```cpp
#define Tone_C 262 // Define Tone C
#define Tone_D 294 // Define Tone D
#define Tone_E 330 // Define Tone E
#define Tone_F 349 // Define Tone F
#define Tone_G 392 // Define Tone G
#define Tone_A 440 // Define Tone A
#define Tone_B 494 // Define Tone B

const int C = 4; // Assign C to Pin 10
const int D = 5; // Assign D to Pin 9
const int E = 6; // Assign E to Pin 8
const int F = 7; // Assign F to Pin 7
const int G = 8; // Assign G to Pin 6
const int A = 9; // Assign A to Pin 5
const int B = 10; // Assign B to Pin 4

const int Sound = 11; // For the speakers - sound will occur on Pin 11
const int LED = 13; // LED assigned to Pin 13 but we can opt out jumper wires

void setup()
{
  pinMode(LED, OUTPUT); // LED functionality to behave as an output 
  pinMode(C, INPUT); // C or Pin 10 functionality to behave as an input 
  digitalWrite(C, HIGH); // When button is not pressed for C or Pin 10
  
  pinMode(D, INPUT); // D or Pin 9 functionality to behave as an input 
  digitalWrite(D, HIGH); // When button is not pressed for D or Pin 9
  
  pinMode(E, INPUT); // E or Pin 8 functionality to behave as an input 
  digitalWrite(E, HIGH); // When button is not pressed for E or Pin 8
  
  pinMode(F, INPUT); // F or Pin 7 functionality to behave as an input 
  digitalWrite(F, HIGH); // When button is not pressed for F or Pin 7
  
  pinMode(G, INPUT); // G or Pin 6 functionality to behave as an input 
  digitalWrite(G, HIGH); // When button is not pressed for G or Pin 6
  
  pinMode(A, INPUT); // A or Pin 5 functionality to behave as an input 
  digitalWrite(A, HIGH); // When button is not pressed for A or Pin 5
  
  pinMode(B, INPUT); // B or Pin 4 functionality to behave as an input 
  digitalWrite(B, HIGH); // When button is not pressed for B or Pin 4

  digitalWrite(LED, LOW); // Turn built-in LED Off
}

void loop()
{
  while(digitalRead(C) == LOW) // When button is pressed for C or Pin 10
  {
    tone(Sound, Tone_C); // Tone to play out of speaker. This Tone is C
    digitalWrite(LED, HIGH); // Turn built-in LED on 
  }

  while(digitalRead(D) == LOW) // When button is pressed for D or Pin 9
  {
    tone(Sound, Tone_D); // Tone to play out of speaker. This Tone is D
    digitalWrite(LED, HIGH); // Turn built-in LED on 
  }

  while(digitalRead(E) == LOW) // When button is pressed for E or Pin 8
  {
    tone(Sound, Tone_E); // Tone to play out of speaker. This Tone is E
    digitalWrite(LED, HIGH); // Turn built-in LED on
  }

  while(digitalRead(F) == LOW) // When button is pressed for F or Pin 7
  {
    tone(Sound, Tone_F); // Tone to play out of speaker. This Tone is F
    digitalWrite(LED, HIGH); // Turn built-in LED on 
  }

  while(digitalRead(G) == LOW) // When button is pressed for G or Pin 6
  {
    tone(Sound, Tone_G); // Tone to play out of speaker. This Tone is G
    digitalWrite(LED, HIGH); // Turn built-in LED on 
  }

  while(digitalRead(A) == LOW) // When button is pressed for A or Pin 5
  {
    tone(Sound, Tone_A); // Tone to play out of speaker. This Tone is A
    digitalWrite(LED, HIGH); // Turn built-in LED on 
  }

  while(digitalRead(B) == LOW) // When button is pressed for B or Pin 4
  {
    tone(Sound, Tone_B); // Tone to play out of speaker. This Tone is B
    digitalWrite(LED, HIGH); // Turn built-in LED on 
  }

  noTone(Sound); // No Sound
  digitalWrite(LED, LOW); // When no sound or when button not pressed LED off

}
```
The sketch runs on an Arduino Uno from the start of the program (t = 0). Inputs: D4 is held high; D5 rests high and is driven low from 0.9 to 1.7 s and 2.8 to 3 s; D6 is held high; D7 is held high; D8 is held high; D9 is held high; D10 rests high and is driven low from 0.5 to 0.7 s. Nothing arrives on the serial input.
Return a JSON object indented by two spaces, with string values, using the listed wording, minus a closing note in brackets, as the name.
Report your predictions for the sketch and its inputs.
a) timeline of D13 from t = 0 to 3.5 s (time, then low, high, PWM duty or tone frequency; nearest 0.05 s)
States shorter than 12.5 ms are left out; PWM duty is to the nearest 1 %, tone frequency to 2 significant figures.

{
  "timeline of D13 from t = 0 to 3.5 s": "0 s low; 0.5 s high; 0.7 s low; 0.9 s high; 1.7 s low; 2.8 s high; 3 s low"
}
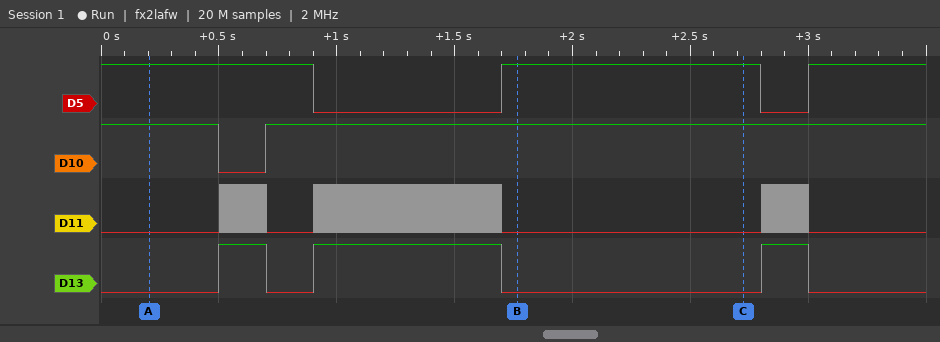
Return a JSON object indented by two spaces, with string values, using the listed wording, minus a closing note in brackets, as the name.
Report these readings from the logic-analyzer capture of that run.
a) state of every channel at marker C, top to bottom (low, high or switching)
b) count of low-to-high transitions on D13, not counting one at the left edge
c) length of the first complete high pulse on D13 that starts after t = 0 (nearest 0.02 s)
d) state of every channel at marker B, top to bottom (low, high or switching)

{
  "state of every channel at marker C, top to bottom": "D5 high, D10 high, D11 low, D13 low",
  "count of low-to-high transitions on D13, not counting one at the left edge": "3",
  "length of the first complete high pulse on D13 that starts after t = 0": "0.20 s",
  "state of every channel at marker B, top to bottom": "D5 high, D10 high, D11 low, D13 low"
}
